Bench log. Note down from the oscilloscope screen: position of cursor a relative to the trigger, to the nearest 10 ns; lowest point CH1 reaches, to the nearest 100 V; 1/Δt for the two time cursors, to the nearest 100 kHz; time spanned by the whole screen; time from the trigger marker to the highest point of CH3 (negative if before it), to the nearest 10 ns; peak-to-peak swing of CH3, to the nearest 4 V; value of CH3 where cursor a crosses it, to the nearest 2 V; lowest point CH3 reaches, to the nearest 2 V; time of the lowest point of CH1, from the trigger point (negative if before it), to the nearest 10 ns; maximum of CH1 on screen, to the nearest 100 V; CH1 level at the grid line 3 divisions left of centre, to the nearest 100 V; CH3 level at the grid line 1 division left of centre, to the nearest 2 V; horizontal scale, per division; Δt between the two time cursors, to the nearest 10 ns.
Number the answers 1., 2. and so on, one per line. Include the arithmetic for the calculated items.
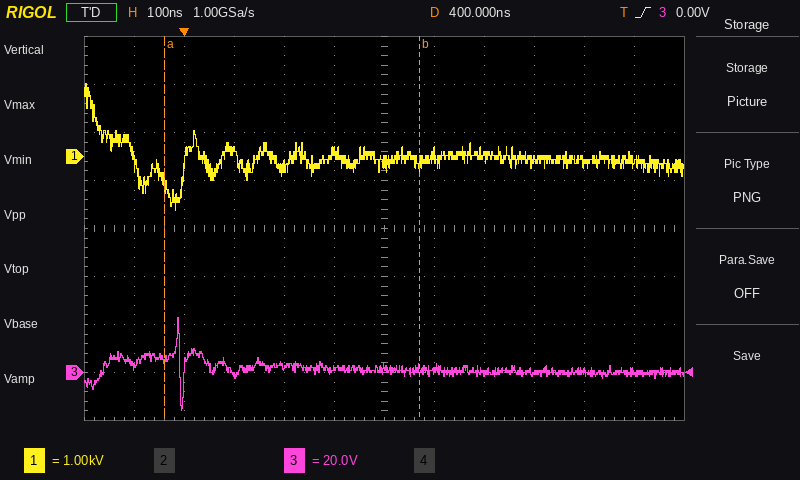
1. -40 ns
2. -1.1 kV
3. 1 / 510 ns ≈ 2.0 MHz
4. 1.2 µs
5. -10 ns
6. 40 V
7. 6 V
8. -16 V
9. -20 ns
10. 1.5 kV
11. 100 V
12. 2 V
13. 100 ns
14. 510 ns
